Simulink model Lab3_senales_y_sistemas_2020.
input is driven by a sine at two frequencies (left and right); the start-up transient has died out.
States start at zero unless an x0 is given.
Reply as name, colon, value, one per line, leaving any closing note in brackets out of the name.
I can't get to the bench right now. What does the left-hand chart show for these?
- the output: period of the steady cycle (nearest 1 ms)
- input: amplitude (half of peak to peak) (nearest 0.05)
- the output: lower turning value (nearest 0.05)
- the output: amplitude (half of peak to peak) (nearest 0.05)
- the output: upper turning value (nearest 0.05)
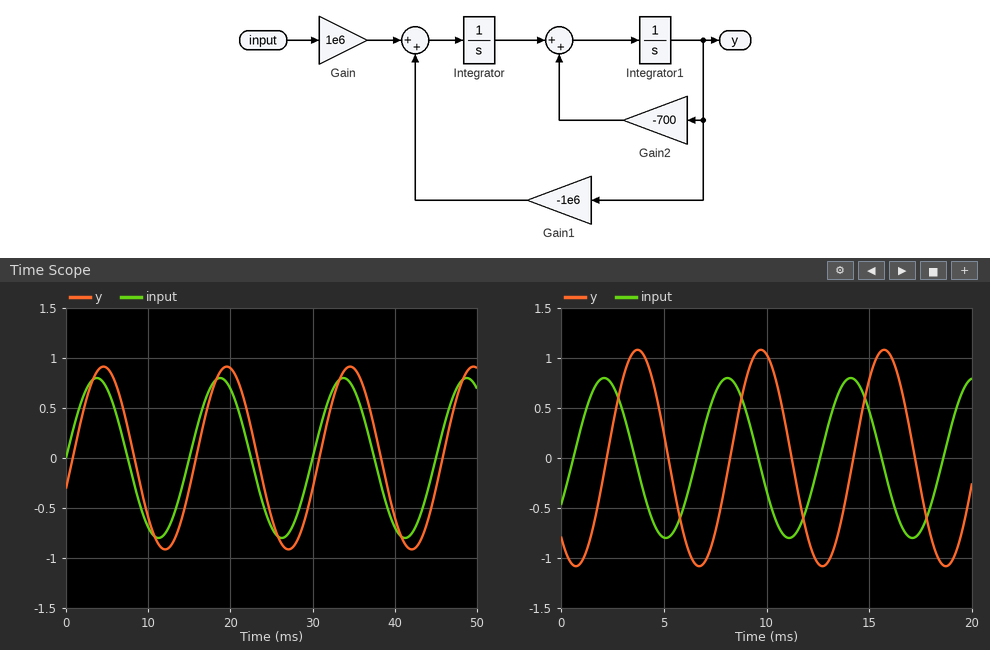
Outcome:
the output: period of the steady cycle: 15 ms
input: amplitude (half of peak to peak): 0.80
the output: lower turning value: -0.90
the output: amplitude (half of peak to peak): 0.90
the output: upper turning value: 0.90
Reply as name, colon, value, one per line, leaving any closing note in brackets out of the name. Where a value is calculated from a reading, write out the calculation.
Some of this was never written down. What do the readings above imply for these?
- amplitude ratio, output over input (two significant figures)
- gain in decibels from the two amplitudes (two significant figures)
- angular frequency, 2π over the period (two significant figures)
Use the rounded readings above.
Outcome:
amplitude ratio, output over input: 0.9 / 0.8 = 1.1
gain in decibels from the two amplitudes: 20 log10(0.9 / 0.8) = 1.0 dB
angular frequency, 2π over the period: 2π / 15 = 0.42 rad/ms
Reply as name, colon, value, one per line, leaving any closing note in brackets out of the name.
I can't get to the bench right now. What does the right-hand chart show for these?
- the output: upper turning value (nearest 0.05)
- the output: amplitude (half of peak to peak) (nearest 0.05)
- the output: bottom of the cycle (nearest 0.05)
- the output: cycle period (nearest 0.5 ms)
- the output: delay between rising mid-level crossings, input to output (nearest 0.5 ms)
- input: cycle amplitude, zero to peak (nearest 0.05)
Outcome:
the output: upper turning value: 1.10
the output: amplitude (half of peak to peak): 1.10
the output: bottom of the cycle: -1.10
the output: cycle period: 6.0 ms
the output: delay between rising mid-level crossings, input to output: 1.5 ms
input: cycle amplitude, zero to peak: 0.80
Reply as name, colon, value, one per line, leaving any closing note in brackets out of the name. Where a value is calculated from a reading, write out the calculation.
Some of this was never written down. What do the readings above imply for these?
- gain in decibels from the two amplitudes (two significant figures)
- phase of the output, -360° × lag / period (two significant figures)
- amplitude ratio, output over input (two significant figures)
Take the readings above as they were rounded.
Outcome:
gain in decibels from the two amplitudes: 20 log10(1.1 / 0.8) = 2.8 dB
phase of the output, -360° × lag / period: -360 × 1.5 / 6 = -90°
amplitude ratio, output over input: 1.1 / 0.8 = 1.4
